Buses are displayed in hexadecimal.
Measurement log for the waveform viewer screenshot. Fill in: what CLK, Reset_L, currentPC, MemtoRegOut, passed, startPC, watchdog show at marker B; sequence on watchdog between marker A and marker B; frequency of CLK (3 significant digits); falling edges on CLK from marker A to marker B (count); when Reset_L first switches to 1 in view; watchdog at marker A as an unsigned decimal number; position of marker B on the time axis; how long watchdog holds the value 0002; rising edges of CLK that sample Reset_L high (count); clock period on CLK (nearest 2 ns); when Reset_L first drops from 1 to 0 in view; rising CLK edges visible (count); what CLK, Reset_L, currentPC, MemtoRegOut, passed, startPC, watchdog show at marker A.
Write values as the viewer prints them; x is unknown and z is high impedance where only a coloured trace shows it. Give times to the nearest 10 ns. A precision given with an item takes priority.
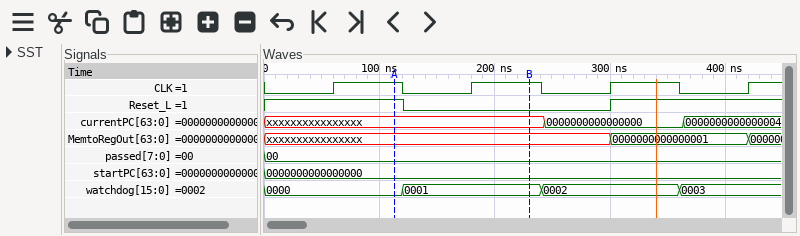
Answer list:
CLK=1, Reset_L=0, currentPC=xxxxxxxxxxxxxxxx, MemtoRegOut=xxxxxxxxxxxxxxxx, passed=00, startPC=0000000000000000, watchdog=0001
0000, 0001
8.33 MHz
1
300 ns
0
230 ns
120 ns
2
120 ns
120 ns
4
CLK=1, Reset_L=1, currentPC=xxxxxxxxxxxxxxxx, MemtoRegOut=xxxxxxxxxxxxxxxx, passed=00, startPC=0000000000000000, watchdog=0000
